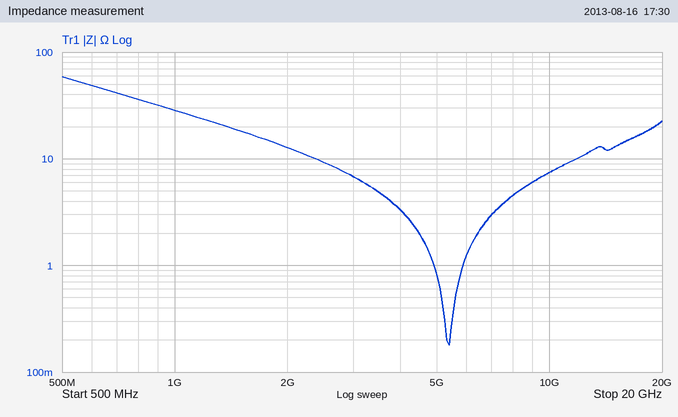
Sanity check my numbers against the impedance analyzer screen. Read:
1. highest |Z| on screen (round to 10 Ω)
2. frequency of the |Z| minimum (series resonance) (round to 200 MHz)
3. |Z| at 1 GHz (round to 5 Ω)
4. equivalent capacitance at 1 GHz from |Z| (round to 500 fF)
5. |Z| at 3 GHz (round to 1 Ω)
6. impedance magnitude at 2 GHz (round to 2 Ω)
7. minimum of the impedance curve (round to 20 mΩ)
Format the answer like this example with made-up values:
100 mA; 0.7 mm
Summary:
60 Ω; 5.4 GHz; 30 Ω; 5.5 pF; 7 Ω; 12 Ω; 180 mΩ
